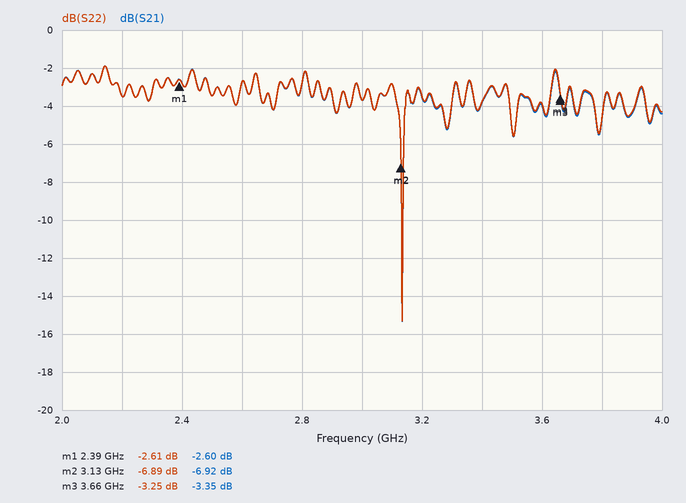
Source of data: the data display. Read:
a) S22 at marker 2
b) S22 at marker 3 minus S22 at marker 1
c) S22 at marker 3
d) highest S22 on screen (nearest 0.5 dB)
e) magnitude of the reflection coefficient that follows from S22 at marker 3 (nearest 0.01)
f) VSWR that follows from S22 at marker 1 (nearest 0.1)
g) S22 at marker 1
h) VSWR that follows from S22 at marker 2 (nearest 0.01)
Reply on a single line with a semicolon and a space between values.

-6.89 dB; -0.64 dB; -3.25 dB; -2.0 dB; 0.69; 6.7; -2.61 dB; 2.65
